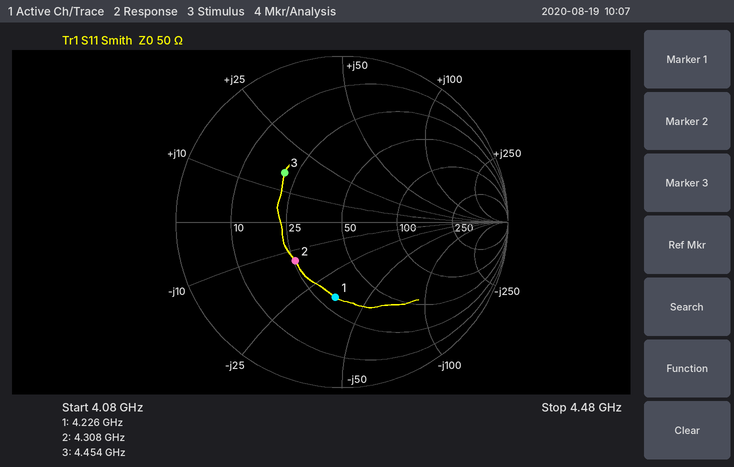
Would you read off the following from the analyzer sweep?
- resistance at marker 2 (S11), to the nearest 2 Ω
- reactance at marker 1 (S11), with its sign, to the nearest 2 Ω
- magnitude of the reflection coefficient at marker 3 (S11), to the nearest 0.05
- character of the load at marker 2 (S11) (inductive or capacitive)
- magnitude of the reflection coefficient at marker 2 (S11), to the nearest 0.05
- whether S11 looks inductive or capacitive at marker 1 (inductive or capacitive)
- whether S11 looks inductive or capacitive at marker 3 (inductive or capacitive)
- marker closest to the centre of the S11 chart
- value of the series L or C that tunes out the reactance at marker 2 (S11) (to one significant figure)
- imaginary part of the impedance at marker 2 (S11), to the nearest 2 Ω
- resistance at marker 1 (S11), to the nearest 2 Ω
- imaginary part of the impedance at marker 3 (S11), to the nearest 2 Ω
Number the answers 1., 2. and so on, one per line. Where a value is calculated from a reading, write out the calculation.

1. 26 Ω
2. -36 Ω
3. 0.45
4. capacitive
5. 0.35
6. capacitive
7. inductive
8. marker 2
9. L = 14 Ω/(2π × 4.308 GHz) ≈ 517 pH, so 500 pH to one significant figure
10. -14 Ω
11. 30 Ω
12. +16 Ω
